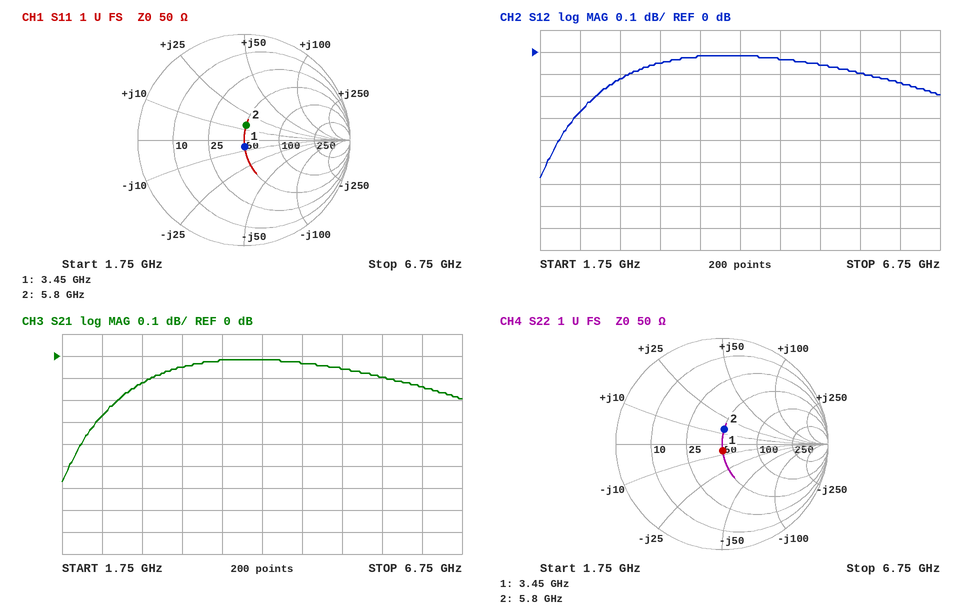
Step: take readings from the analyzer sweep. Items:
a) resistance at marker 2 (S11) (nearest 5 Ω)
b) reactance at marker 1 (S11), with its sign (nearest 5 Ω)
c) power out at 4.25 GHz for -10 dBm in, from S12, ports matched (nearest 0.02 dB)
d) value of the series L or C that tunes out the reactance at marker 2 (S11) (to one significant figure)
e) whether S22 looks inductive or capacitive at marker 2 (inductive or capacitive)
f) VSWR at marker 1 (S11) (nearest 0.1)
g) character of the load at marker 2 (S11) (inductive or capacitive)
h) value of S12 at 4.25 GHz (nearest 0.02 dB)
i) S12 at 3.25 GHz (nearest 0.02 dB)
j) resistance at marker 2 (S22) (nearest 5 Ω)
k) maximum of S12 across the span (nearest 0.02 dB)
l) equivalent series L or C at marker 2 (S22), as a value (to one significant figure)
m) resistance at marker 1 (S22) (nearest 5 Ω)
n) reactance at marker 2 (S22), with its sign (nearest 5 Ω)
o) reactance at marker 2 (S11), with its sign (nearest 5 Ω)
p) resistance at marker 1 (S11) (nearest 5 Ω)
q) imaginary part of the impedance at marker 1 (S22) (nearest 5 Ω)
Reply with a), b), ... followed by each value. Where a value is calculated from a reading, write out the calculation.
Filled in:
a) 50 Ω
b) -5 Ω
c) -10 dBm + (-0.02 dB) = -10.02 dBm
d) C = 1/(2π × 5.8 GHz × 15 Ω) ≈ 2 pF
e) inductive
f) 1.1
g) inductive
h) -0.02 dB
i) -0.06 dB
j) 50 Ω
k) -0.02 dB
l) L = 15 Ω/(2π × 5.8 GHz) ≈ 412 pH, so 400 pH to one significant figure
m) 50 Ω
n) +15 Ω
o) +15 Ω
p) 50 Ω
q) -5 Ω
